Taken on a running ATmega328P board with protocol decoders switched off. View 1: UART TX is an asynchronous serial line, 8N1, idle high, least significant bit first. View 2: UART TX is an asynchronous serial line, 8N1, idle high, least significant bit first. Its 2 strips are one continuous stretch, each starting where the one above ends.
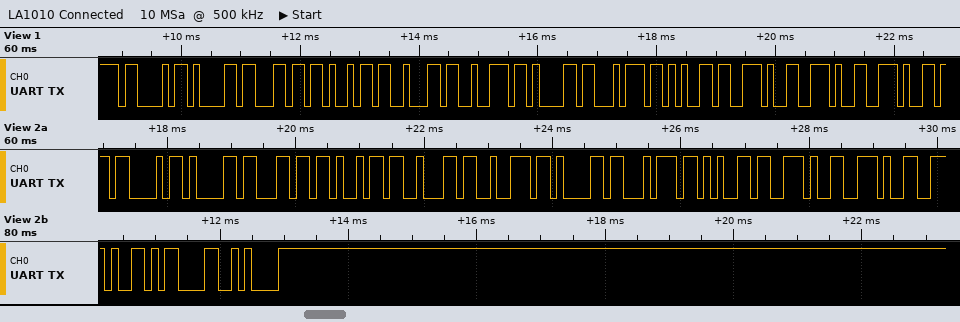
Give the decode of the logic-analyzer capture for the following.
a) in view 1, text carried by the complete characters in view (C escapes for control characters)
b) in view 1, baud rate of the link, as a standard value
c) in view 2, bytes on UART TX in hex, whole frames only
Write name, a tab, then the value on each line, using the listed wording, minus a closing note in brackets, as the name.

in view 1, text carried by the complete characters in view	"Calibrate..."
in view 1, baud rate of the link, as a standard value	9600 baud
in view 2, bytes on UART TX in hex, whole frames only	0x43 0x61 0x6C 0x69 0x62 0x72 0x61 0x74 0x65 0x2E 0x2E 0x2E 0x0D 0x0A
